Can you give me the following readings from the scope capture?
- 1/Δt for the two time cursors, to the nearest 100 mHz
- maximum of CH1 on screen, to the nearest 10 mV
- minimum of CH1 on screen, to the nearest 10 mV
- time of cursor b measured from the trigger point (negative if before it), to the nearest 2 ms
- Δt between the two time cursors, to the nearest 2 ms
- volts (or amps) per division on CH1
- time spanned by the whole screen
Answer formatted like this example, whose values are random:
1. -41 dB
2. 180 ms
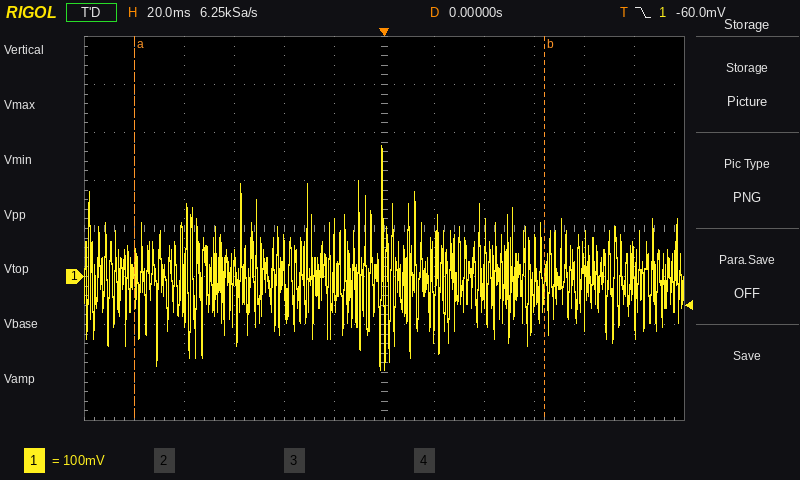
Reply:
1. 6.1 Hz
2. 270 mV
3. -190 mV
4. +64 ms
5. 164 ms
6. 100 mV
7. 240 ms
